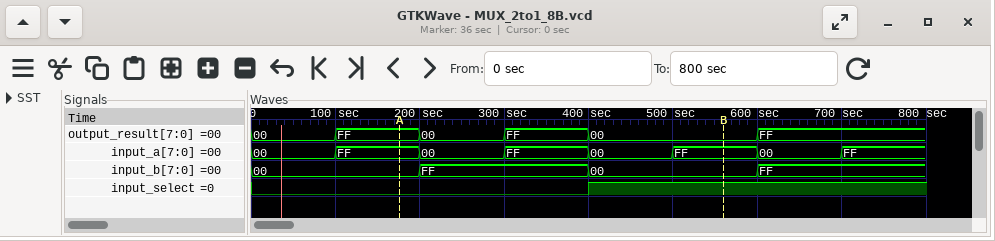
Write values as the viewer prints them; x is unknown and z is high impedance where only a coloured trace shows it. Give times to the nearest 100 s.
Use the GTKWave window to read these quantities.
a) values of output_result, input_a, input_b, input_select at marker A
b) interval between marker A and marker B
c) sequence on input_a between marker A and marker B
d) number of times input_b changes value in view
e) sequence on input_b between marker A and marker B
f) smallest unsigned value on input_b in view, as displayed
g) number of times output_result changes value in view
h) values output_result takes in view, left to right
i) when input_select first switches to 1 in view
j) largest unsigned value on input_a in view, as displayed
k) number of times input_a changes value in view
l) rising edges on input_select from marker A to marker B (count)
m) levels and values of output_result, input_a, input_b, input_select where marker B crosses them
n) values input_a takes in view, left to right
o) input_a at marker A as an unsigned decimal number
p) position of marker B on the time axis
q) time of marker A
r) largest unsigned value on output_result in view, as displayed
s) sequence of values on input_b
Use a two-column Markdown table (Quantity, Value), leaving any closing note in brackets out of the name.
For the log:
| Quantity | Value |
|---|---|
| values of output_result, input_a, input_b, input_select at marker A | output_result=FF, input_a=FF, input_b=00, input_select=0 |
| interval between marker A and marker B | 400 s |
| sequence on input_a between marker A and marker B | FF, 00, FF, 00, FF |
| number of times input_b changes value in view | 3 |
| sequence on input_b between marker A and marker B | 00, FF, 00 |
| smallest unsigned value on input_b in view, as displayed | 00 |
| number of times output_result changes value in view | 5 |
| values output_result takes in view, left to right | 00, FF, 00, FF, 00, FF |
| when input_select first switches to 1 in view | 400 s |
| largest unsigned value on input_a in view, as displayed | FF |
| number of times input_a changes value in view | 7 |
| rising edges on input_select from marker A to marker B | 1 |
| levels and values of output_result, input_a, input_b, input_select where marker B crosses them | output_result=00, input_a=FF, input_b=00, input_select=1 |
| values input_a takes in view, left to right | 00, FF, 00, FF, 00, FF, 00, FF |
| input_a at marker A as an unsigned decimal number | 255 |
| position of marker B on the time axis | 600 s |
| time of marker A | 200 s |
| largest unsigned value on output_result in view, as displayed | FF |
| sequence of values on input_b | 00, FF, 00, FF |
